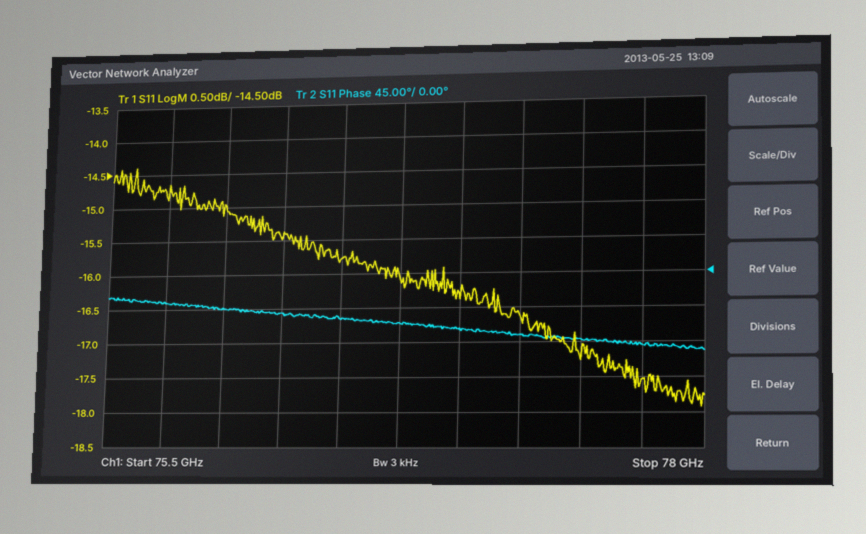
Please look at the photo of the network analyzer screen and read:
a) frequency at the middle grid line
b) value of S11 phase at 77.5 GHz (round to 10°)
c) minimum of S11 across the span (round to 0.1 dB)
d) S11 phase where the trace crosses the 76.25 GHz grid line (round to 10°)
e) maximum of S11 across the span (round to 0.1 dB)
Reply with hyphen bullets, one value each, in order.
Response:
- 76.75 GHz
- -90°
- -17.9 dB
- -50°
- -14.4 dB
